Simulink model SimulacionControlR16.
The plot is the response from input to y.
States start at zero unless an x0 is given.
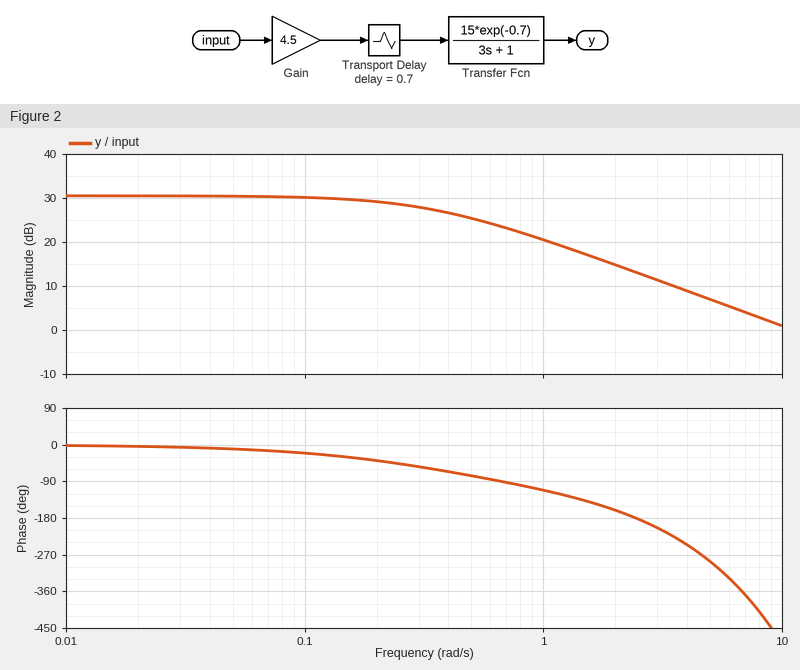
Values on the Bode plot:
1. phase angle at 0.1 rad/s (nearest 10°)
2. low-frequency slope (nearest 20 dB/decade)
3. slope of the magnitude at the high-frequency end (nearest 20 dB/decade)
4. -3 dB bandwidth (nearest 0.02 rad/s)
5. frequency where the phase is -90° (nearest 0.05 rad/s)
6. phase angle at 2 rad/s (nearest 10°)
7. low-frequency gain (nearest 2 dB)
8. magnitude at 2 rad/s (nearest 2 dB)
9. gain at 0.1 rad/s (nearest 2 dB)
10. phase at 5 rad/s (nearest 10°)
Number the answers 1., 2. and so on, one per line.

1. -20°
2. 0 dB/decade
3. -20 dB/decade
4. 0.34 rad/s
5. 0.65 rad/s
6. -160°
7. 30 dB
8. 14 dB
9. 30 dB
10. -290°
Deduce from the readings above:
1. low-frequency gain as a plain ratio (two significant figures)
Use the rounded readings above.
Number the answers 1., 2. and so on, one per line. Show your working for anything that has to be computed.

1. 10^(30 / 20) = 32
